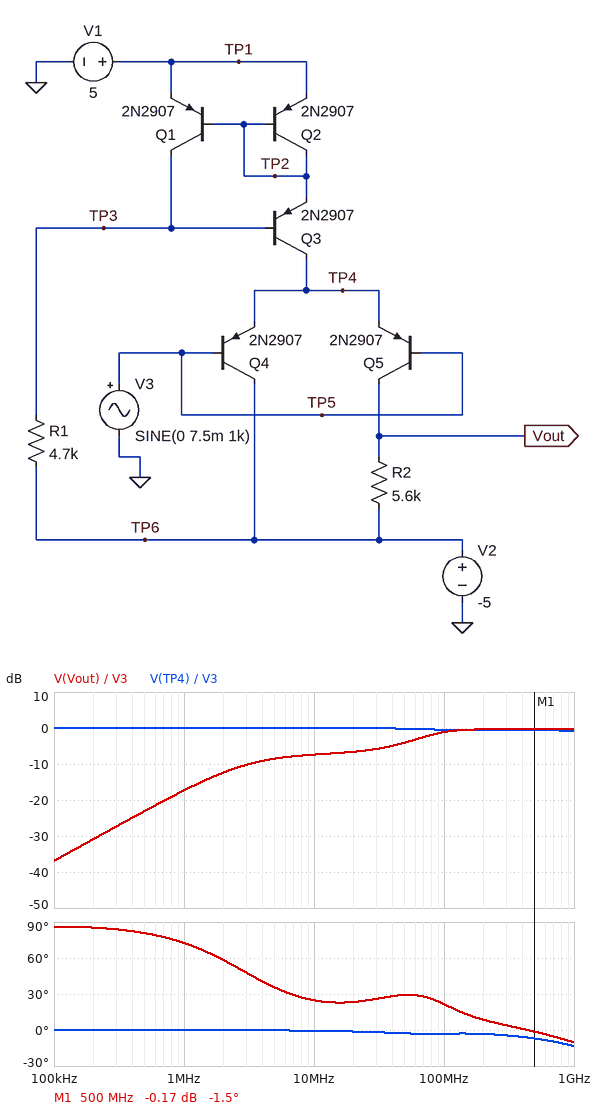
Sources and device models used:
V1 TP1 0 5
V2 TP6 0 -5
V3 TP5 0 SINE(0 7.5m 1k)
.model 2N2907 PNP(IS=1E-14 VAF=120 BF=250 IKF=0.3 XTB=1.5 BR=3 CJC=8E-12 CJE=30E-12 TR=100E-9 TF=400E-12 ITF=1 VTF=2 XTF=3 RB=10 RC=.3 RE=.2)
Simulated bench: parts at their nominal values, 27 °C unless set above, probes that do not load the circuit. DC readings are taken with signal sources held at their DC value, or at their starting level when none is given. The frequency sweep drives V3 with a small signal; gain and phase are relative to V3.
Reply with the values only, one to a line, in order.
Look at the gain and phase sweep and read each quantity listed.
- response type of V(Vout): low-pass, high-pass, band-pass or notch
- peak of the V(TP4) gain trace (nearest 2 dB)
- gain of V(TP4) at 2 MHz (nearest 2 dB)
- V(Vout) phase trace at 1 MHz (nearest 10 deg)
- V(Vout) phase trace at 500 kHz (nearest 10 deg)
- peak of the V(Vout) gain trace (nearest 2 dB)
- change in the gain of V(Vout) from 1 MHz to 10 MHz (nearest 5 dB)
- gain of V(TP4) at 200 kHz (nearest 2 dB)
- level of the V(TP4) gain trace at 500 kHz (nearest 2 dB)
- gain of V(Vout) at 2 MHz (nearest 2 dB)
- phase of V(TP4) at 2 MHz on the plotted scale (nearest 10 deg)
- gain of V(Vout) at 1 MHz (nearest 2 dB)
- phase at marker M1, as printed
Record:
high-pass
0 dB
0 dB
70 deg
80 deg
0 dB
10 dB
0 dB
0 dB
-12 dB
0 deg
-18 dB
-1.5 deg
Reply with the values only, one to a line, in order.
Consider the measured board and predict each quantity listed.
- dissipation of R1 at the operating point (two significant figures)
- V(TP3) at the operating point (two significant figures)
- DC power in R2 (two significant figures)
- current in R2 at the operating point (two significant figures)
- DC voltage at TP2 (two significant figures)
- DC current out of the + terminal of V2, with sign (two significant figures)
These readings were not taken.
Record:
16 mW
3.7 V
4.5 mW
890 µA
4.3 V
-3.7 mA
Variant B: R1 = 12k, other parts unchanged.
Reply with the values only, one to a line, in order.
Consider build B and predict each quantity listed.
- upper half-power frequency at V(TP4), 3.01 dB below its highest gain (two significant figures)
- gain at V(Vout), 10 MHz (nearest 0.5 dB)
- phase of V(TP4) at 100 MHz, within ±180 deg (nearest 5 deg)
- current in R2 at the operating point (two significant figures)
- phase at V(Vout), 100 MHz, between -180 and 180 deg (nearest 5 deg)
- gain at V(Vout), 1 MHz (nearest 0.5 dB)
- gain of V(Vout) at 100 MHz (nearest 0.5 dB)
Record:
3.5 GHz
-12.5 dB
0 deg
360 µA
15 deg
-43.0 dB
0 dB
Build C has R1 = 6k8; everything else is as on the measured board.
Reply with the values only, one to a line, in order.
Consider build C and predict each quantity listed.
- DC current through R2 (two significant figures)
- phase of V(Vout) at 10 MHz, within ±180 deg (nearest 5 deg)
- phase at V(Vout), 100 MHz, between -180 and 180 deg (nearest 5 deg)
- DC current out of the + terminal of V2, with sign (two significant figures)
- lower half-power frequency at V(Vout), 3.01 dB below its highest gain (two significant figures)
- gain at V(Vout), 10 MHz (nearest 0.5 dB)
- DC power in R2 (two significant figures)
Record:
620 µA
55 deg
25 deg
-2.5 mA
49 MHz
-13.5 dB
2.2 mW
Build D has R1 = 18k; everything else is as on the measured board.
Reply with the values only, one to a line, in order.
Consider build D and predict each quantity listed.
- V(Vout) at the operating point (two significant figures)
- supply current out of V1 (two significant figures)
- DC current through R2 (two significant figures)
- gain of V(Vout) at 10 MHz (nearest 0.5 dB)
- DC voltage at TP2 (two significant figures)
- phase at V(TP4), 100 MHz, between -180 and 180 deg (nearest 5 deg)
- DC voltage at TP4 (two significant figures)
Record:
-3.7 V
970 µA
240 µA
-9.5 dB
4.4 V
0 deg
620 mV
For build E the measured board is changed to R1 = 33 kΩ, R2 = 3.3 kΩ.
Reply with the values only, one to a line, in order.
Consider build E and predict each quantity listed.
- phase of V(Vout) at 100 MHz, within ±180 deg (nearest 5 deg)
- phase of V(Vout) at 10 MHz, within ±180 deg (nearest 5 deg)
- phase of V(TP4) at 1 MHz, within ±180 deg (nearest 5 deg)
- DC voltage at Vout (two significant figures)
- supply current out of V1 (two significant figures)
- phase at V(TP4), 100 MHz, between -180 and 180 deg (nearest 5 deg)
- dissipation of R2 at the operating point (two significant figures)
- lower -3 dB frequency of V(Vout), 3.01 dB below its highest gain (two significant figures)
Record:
10 deg
115 deg
0 deg
-4.6 V
530 µA
0 deg
57 µW
15 MHz
